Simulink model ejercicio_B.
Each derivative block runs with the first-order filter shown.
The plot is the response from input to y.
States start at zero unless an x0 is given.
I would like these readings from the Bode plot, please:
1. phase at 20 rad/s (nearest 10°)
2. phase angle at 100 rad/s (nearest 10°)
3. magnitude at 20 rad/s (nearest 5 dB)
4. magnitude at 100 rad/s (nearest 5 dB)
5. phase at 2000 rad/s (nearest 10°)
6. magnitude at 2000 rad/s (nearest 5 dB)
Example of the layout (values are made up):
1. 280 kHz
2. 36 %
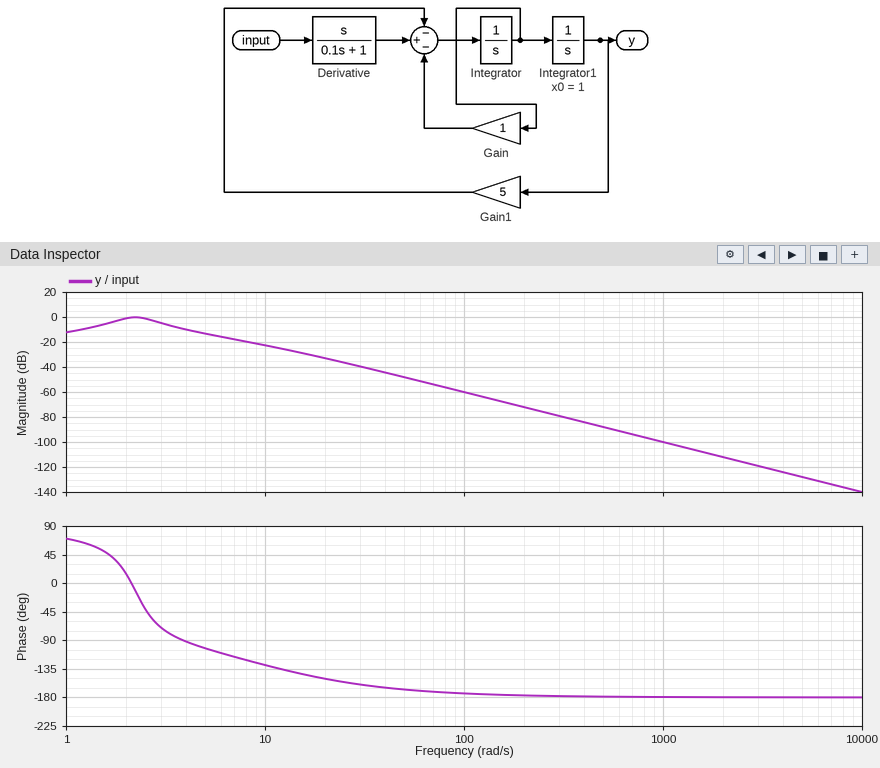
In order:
1. -150°
2. -170°
3. -35 dB
4. -60 dB
5. -180°
6. -110 dB
